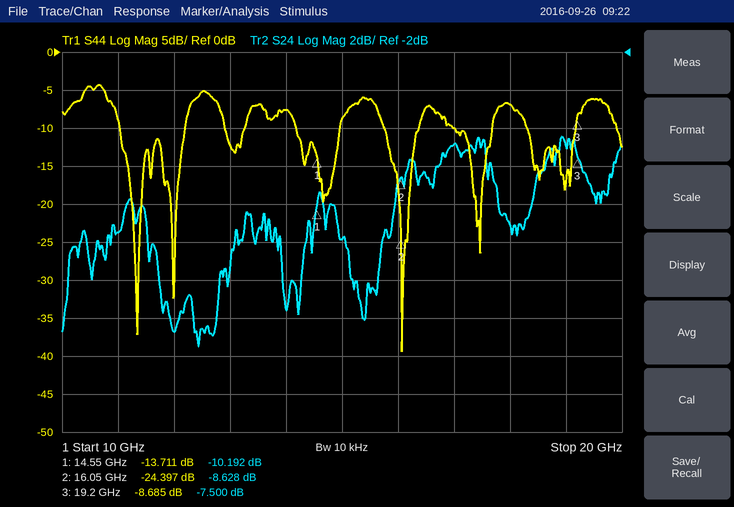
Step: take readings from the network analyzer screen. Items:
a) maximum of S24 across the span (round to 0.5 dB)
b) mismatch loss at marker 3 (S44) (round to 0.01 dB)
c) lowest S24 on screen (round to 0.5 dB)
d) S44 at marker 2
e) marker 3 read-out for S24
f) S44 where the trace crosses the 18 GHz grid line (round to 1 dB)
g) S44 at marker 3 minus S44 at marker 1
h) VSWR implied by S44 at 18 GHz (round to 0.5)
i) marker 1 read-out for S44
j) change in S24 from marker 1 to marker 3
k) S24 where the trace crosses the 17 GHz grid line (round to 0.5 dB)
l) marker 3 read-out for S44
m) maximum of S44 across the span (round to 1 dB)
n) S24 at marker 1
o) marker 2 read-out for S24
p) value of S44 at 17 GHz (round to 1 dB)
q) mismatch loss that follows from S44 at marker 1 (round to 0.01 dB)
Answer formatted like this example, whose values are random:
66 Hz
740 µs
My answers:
-6.5 dB
0.63 dB
-17.5 dB
-24.397 dB
-7.500 dB
-7 dB
5.026 dB
2.5
-13.711 dB
2.692 dB
-7.0 dB
-8.685 dB
-4 dB
-10.192 dB
-8.628 dB
-10 dB
0.19 dB
